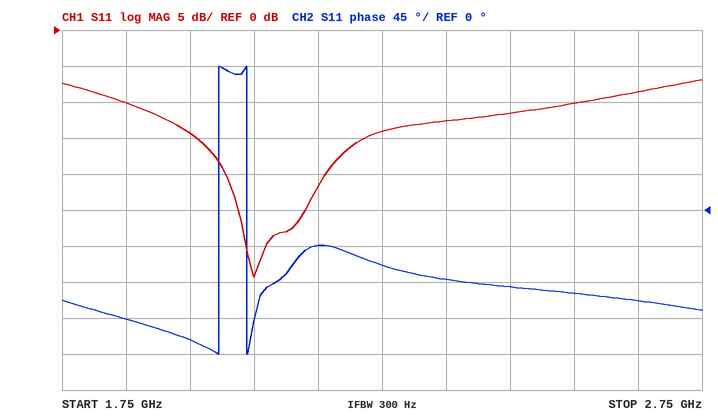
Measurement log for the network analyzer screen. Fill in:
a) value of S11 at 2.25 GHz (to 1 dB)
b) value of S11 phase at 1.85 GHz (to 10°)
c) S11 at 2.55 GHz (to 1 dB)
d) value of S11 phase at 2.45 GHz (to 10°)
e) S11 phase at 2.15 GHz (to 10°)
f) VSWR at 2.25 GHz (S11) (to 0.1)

-14 dB
-140°
-10 dB
-100°
-40°
1.5
